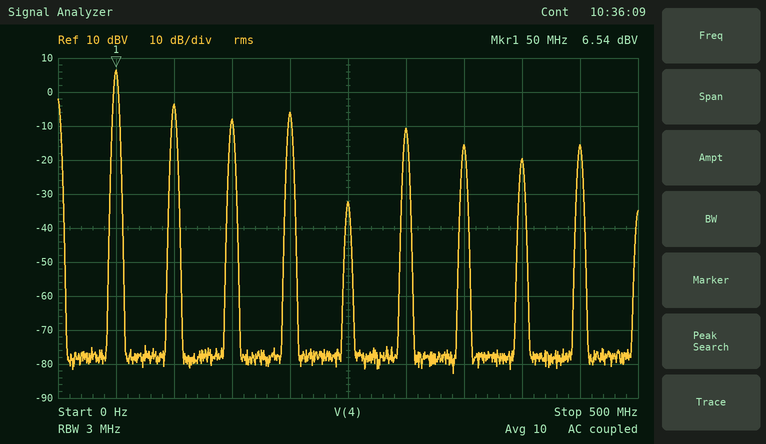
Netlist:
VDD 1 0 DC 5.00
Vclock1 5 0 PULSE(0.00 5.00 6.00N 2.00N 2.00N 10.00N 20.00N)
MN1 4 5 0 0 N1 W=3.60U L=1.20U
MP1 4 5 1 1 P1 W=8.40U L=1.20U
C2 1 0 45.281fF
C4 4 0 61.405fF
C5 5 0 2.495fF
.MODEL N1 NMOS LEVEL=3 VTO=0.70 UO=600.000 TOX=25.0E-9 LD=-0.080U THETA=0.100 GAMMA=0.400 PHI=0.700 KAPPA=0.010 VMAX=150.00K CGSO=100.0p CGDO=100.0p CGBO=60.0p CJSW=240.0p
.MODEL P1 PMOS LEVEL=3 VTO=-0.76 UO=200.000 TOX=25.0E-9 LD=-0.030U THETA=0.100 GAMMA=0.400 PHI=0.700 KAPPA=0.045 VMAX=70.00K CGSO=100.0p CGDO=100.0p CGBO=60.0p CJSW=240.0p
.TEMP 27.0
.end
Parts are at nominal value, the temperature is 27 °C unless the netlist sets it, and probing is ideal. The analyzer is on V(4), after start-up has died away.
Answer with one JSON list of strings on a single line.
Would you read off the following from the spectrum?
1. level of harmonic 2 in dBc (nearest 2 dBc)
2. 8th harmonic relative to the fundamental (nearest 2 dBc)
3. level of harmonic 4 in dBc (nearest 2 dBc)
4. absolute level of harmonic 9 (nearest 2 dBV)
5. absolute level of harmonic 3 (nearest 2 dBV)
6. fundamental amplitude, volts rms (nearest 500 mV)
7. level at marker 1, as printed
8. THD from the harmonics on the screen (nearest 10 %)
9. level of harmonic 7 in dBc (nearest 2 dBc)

["-10 dBc", "-26 dBc", "-12 dBc", "-16 dBV", "-8 dBV", "2.0 V", "6.54 dBV", "50 %", "-22 dBc"]
